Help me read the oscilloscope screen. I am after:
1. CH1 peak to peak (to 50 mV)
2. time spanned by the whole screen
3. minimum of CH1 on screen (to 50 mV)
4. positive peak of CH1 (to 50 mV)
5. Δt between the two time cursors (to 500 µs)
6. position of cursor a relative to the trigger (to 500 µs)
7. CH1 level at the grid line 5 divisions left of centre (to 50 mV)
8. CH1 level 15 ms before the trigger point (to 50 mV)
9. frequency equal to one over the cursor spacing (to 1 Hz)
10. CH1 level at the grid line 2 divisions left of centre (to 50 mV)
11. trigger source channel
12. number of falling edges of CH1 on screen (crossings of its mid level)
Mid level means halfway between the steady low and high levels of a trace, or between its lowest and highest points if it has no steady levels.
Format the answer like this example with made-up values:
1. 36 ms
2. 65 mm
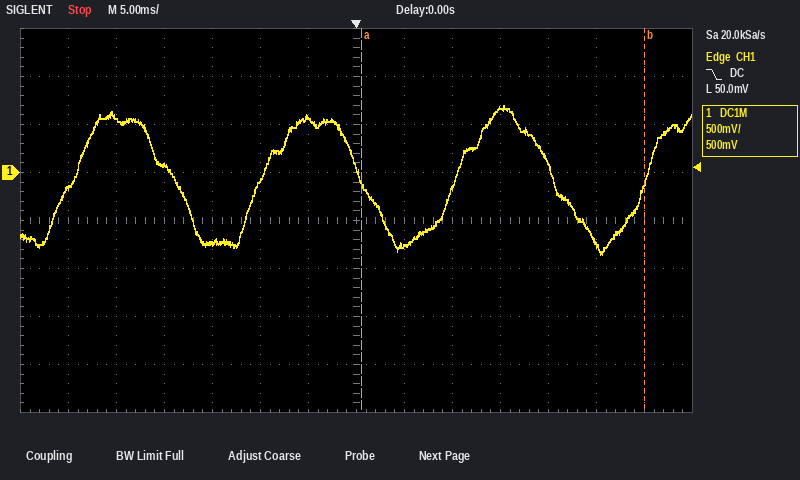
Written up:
1. 1.55 V
2. 70 ms
3. -850 mV
4. 700 mV
5. 29.5 ms
6. +500 µs
7. 550 mV
8. -750 mV
9. 34 Hz
10. -100 mV
11. CH1
12. 3
